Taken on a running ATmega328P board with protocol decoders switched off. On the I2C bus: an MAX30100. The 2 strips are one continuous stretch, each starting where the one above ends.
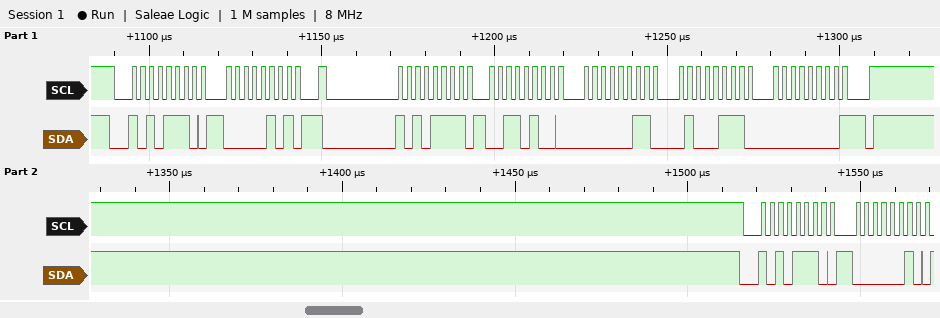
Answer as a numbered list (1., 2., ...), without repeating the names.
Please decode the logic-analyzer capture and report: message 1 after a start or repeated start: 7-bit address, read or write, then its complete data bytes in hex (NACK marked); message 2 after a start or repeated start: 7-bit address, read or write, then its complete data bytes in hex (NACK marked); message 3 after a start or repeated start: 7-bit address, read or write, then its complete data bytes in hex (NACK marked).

1. 0x57 write: 05
2. 0x57 read: 34 03 47 00 NACK
3. 0x57 write: 02
